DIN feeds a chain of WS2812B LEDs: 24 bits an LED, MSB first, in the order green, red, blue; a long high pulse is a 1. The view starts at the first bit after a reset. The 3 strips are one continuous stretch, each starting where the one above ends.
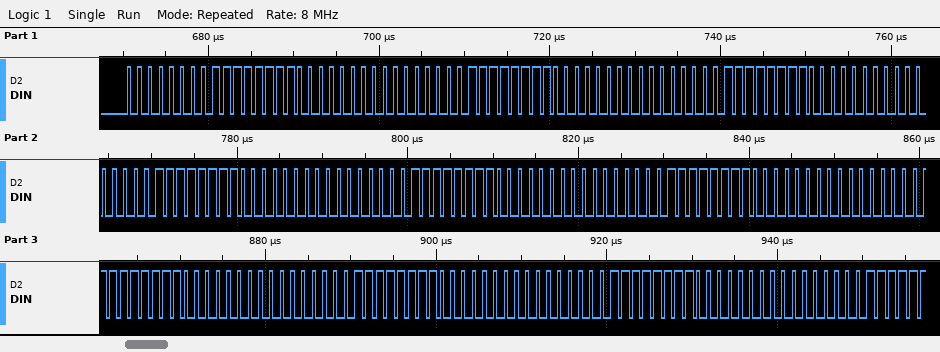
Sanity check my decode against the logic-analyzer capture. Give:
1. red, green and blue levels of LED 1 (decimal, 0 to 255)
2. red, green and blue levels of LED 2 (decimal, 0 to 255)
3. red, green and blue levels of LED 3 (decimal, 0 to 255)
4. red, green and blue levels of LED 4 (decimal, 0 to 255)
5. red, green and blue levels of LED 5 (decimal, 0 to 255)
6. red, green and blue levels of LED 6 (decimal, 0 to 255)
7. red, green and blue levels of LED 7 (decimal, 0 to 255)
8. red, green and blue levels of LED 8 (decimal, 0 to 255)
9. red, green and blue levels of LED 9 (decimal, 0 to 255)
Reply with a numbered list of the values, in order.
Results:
1. 255, 0, 0
2. 255, 0, 0
3. 255, 0, 0
4. 255, 0, 0
5. 255, 0, 0
6. 255, 0, 0
7. 255, 0, 0
8. 255, 0, 0
9. 255, 0, 0
